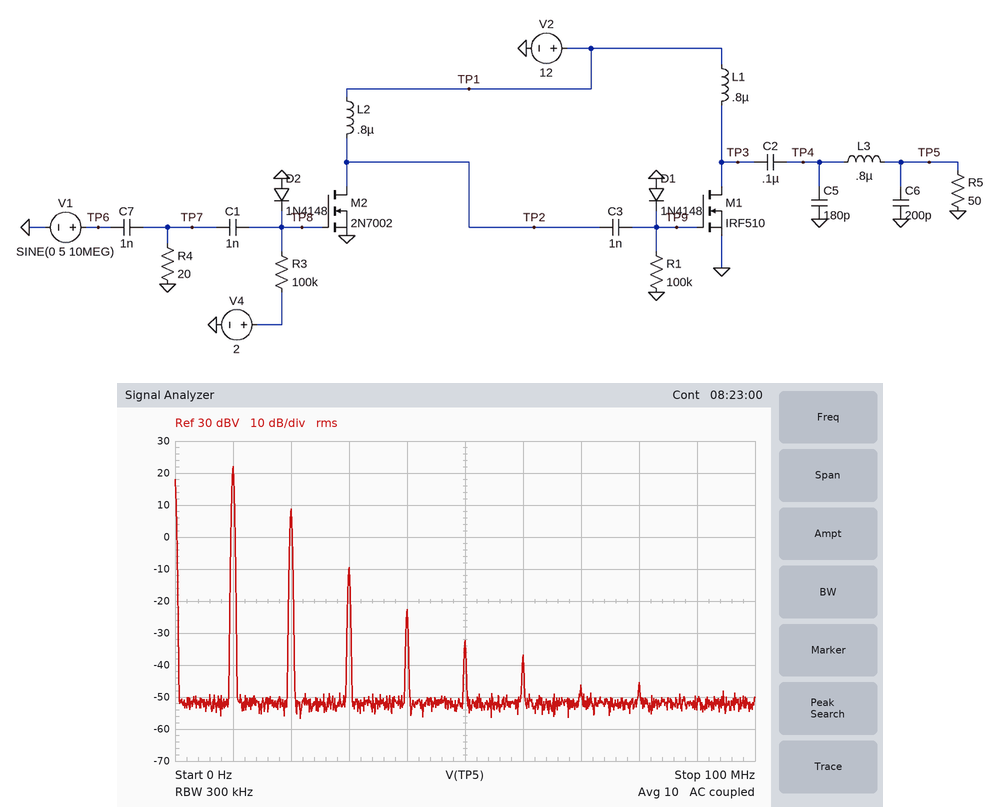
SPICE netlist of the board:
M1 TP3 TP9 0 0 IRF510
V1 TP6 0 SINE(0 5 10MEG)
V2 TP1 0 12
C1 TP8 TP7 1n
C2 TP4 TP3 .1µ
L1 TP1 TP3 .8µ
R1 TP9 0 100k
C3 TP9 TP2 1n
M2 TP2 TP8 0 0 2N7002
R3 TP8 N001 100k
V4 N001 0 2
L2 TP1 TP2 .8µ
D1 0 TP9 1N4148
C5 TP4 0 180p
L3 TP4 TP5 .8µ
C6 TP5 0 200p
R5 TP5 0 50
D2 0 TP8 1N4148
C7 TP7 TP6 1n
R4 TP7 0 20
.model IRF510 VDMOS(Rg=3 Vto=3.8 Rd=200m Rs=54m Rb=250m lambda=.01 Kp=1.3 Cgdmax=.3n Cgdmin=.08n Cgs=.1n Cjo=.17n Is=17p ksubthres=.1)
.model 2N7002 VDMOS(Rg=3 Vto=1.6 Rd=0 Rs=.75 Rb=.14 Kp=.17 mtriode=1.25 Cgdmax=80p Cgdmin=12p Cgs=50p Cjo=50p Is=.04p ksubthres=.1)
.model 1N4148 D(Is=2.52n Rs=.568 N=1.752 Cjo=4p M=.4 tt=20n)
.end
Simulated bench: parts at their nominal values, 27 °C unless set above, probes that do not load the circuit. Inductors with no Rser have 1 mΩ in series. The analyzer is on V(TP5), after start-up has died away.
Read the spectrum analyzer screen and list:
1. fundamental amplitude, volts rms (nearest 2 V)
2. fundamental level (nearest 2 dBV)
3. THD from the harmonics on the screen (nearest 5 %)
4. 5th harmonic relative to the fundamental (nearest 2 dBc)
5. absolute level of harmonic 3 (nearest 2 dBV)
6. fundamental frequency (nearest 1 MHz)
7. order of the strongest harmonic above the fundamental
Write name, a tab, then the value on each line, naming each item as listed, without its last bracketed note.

fundamental amplitude, volts rms	12 V
fundamental level	22 dBV
THD from the harmonics on the screen	20 %
5th harmonic relative to the fundamental	-54 dBc
absolute level of harmonic 3	-10 dBV
fundamental frequency	10 MHz
order of the strongest harmonic above the fundamental	2
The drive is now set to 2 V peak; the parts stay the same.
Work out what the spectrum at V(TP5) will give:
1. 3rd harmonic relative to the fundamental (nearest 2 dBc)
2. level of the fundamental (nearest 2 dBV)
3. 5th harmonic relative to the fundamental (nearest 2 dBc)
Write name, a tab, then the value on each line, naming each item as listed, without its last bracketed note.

3rd harmonic relative to the fundamental	-32 dBc
level of the fundamental	22 dBV
5th harmonic relative to the fundamental	-58 dBc
